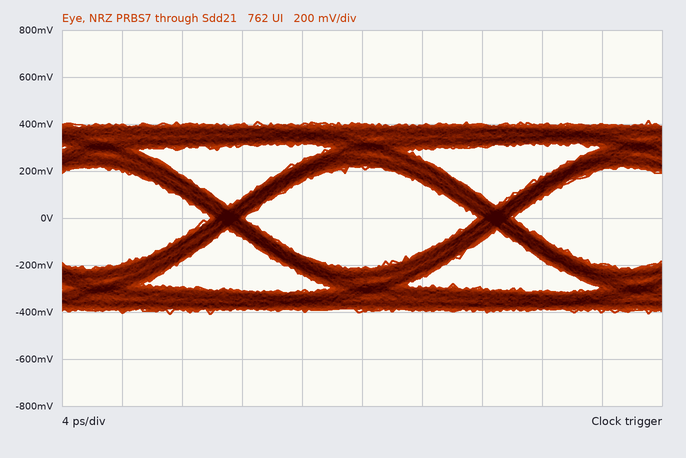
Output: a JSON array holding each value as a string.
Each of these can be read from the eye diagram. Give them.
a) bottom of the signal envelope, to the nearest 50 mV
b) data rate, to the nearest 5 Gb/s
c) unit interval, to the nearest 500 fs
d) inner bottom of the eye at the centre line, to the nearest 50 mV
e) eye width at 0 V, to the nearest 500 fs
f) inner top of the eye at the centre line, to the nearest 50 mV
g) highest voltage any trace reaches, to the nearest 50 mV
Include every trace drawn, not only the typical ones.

["-400 mV", "55 Gb/s", "18.0 ps", "-200 mV", "15.5 ps", "200 mV", "400 mV"]
